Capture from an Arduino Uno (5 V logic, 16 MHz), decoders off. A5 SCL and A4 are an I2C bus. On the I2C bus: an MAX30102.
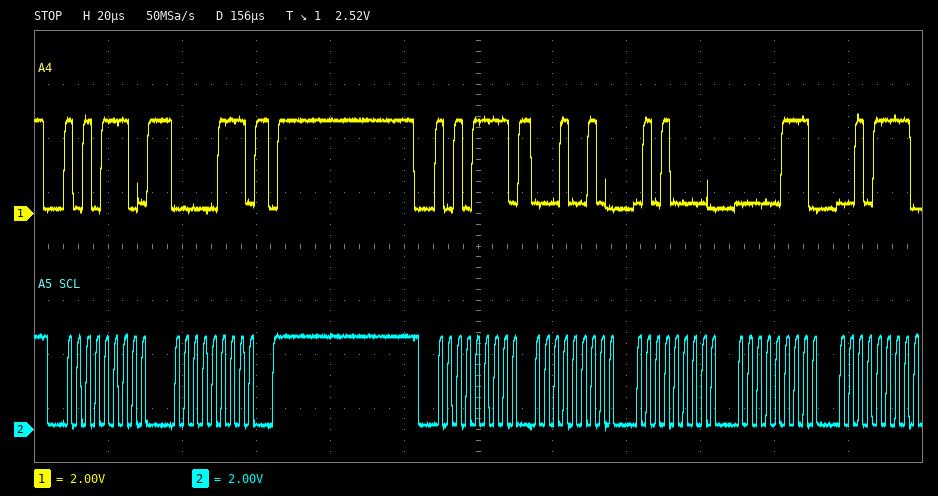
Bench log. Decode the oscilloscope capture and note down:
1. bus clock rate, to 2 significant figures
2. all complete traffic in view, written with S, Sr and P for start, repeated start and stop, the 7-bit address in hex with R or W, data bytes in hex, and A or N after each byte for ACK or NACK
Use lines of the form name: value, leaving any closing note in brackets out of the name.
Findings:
bus clock rate, to 2 significant figures: 400 kHz
all complete traffic in view, written with S, Sr and P for start, repeated start and stop, the 7-bit address in hex with R or W, data bytes in hex, and A or N after each byte for ACK or NACK: S 57W A 07 A P S 57R A 12 A 50 A 07 A 2F A
